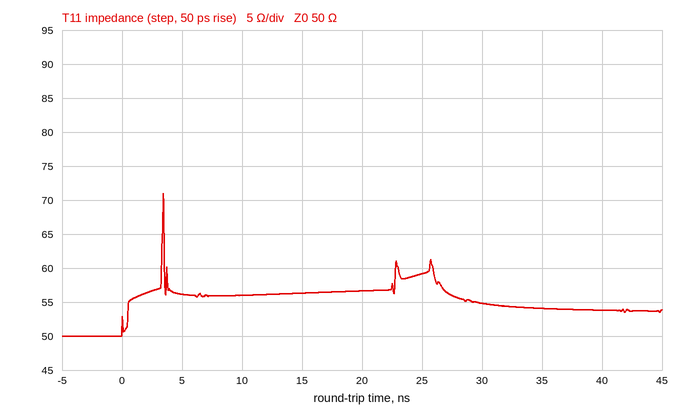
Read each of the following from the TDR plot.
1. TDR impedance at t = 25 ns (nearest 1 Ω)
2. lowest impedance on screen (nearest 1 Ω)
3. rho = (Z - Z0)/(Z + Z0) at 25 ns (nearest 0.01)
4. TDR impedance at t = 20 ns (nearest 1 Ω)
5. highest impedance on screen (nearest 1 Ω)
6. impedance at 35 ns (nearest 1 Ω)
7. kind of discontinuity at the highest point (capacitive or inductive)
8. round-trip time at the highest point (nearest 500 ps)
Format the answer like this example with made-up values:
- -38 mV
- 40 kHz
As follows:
- 59 Ω
- 50 Ω
- +0.08
- 57 Ω
- 71 Ω
- 54 Ω
- inductive
- 3.5 ns
